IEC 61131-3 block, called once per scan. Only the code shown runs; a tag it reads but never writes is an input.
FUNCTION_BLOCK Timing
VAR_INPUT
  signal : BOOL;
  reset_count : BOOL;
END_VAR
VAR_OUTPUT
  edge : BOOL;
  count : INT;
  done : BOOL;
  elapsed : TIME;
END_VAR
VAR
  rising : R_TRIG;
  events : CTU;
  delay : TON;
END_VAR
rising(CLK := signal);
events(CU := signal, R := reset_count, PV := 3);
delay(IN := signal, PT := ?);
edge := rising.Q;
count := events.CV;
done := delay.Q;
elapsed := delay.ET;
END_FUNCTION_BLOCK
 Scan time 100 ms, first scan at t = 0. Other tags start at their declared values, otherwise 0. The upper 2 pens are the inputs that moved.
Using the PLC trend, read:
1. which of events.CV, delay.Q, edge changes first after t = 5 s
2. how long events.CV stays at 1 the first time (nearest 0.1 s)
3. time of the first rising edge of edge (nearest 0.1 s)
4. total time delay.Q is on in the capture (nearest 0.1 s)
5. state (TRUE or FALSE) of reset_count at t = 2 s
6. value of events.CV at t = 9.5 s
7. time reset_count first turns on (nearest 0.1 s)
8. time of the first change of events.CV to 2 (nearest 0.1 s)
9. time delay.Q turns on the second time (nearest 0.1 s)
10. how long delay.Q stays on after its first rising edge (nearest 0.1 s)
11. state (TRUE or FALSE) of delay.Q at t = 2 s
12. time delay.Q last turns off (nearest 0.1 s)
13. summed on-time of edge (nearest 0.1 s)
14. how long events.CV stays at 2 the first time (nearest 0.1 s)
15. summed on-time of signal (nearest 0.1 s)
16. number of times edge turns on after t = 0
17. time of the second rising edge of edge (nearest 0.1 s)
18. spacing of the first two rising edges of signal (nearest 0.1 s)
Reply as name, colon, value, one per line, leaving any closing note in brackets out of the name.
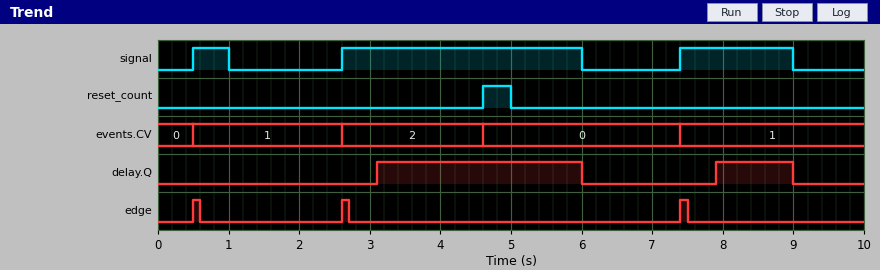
which of events.CV, delay.Q, edge changes first after t = 5 s: delay.Q
how long events.CV stays at 1 the first time: 2.1 s
time of the first rising edge of edge: 0.5 s
total time delay.Q is on in the capture: 4.0 s
state (TRUE or FALSE) of reset_count at t = 2 s: FALSE
value of events.CV at t = 9.5 s: 1
time reset_count first turns on: 4.6 s
time of the first change of events.CV to 2: 2.6 s
time delay.Q turns on the second time: 7.9 s
how long delay.Q stays on after its first rising edge: 2.9 s
state (TRUE or FALSE) of delay.Q at t = 2 s: FALSE
time delay.Q last turns off: 9.0 s
summed on-time of edge: 0.3 s
how long events.CV stays at 2 the first time: 2.0 s
summed on-time of signal: 5.5 s
number of times edge turns on after t = 0: 3
time of the second rising edge of edge: 2.6 s
spacing of the first two rising edges of signal: 2.1 s
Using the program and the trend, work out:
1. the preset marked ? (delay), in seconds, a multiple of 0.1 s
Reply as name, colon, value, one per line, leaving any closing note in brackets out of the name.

the preset marked ? (delay), in seconds, a multiple of 0.1 s: 0.5 s
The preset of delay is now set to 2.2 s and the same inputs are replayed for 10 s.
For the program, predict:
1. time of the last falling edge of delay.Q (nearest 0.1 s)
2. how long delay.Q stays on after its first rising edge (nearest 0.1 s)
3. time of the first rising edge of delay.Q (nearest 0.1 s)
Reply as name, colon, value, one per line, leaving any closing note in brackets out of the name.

time of the last falling edge of delay.Q: 6.0 s
how long delay.Q stays on after its first rising edge: 1.2 s
time of the first rising edge of delay.Q: 4.8 s
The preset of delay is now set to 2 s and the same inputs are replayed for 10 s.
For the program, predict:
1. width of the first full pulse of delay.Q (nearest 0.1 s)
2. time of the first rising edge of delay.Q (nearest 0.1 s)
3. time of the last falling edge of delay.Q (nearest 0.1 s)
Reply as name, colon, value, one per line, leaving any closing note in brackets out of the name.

width of the first full pulse of delay.Q: 1.4 s
time of the first rising edge of delay.Q: 4.6 s
time of the last falling edge of delay.Q: 6.0 s
